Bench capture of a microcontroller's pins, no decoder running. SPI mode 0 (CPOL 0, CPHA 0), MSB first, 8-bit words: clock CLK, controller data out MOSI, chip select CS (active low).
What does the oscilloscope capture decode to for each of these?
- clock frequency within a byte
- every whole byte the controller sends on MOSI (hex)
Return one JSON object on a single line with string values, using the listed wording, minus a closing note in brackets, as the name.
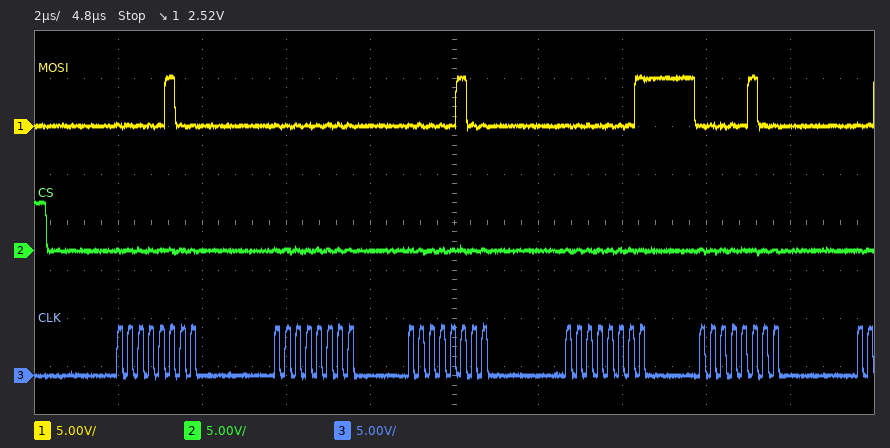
{"clock frequency within a byte": "4 MHz", "every whole byte the controller sends on MOSI": "0x04 0x00 0x04 0x01 0x04"}
